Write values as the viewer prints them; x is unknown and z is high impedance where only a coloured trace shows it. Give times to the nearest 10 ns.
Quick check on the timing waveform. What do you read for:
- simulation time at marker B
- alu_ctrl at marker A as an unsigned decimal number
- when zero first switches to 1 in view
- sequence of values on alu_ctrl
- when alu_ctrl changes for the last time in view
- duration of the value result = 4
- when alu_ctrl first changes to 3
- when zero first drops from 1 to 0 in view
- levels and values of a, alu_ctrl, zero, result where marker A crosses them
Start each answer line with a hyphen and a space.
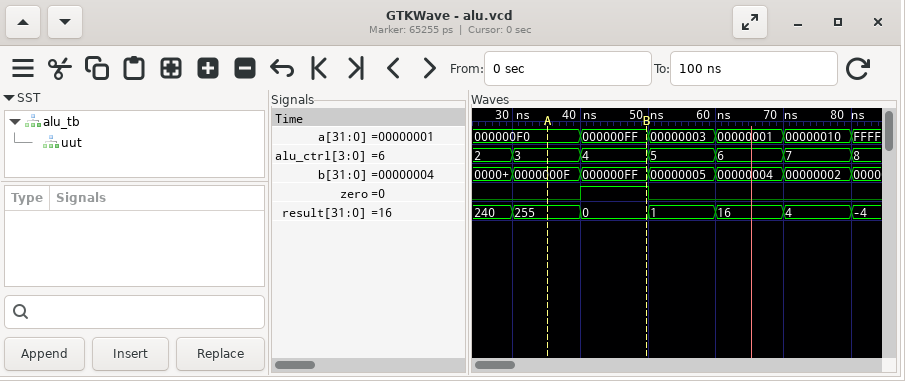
- 50 ns
- 3
- 40 ns
- 2, 3, 4, 5, 6, 7, 8
- 80 ns
- 10 ns
- 30 ns
- 50 ns
- a=000000F0, alu_ctrl=3, zero=0, result=255
